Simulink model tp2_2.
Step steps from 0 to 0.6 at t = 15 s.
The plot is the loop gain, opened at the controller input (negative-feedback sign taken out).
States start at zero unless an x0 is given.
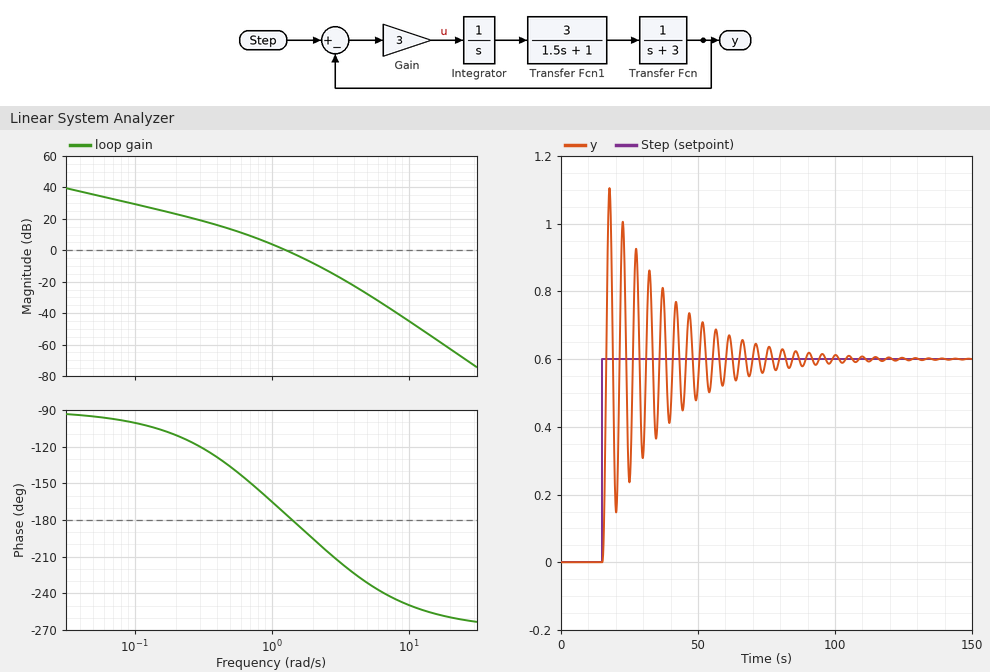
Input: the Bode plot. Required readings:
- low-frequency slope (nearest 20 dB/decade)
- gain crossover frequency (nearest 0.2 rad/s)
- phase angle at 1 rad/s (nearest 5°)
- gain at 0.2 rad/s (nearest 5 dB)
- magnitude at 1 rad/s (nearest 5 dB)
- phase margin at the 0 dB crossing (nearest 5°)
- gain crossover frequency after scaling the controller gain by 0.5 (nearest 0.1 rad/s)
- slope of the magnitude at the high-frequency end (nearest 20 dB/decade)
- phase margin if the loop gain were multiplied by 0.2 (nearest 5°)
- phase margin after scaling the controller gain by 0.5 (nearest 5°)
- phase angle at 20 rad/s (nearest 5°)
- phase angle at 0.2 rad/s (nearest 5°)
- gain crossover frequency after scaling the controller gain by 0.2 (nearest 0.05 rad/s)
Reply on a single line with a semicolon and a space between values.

-20 dB/decade; 1.2 rad/s; -165°; 25 dB; 5 dB; 5°; 0.9 rad/s; -60 dB/decade; 45°; 20°; -260°; -110°; 0.50 rad/s
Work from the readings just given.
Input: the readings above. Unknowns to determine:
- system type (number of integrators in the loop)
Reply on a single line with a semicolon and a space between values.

1
